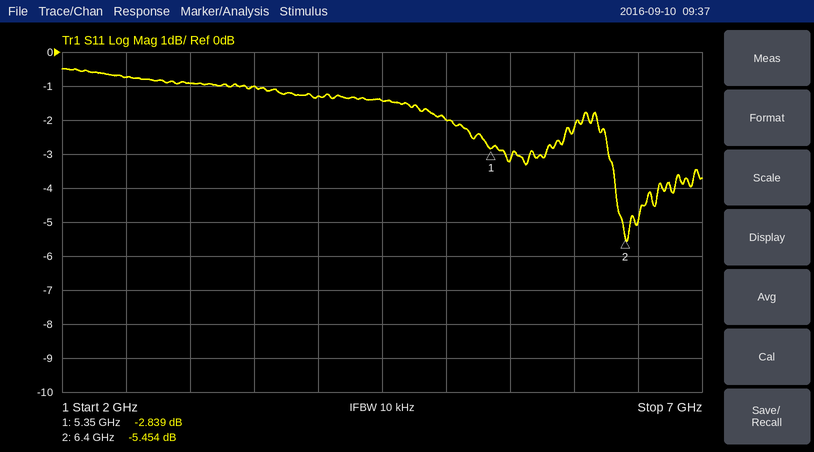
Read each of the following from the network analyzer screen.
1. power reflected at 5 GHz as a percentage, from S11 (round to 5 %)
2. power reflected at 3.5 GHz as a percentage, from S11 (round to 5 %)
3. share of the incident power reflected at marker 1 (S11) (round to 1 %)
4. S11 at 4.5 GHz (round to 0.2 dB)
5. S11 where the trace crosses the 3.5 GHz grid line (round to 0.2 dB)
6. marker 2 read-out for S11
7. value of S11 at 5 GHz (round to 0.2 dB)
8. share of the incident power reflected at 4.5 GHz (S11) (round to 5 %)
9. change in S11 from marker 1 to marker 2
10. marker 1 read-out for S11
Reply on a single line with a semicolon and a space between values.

65 %; 80 %; 52 %; -1.4 dB; -1.0 dB; -5.454 dB; -2.0 dB; 70 %; -2.615 dB; -2.839 dB
